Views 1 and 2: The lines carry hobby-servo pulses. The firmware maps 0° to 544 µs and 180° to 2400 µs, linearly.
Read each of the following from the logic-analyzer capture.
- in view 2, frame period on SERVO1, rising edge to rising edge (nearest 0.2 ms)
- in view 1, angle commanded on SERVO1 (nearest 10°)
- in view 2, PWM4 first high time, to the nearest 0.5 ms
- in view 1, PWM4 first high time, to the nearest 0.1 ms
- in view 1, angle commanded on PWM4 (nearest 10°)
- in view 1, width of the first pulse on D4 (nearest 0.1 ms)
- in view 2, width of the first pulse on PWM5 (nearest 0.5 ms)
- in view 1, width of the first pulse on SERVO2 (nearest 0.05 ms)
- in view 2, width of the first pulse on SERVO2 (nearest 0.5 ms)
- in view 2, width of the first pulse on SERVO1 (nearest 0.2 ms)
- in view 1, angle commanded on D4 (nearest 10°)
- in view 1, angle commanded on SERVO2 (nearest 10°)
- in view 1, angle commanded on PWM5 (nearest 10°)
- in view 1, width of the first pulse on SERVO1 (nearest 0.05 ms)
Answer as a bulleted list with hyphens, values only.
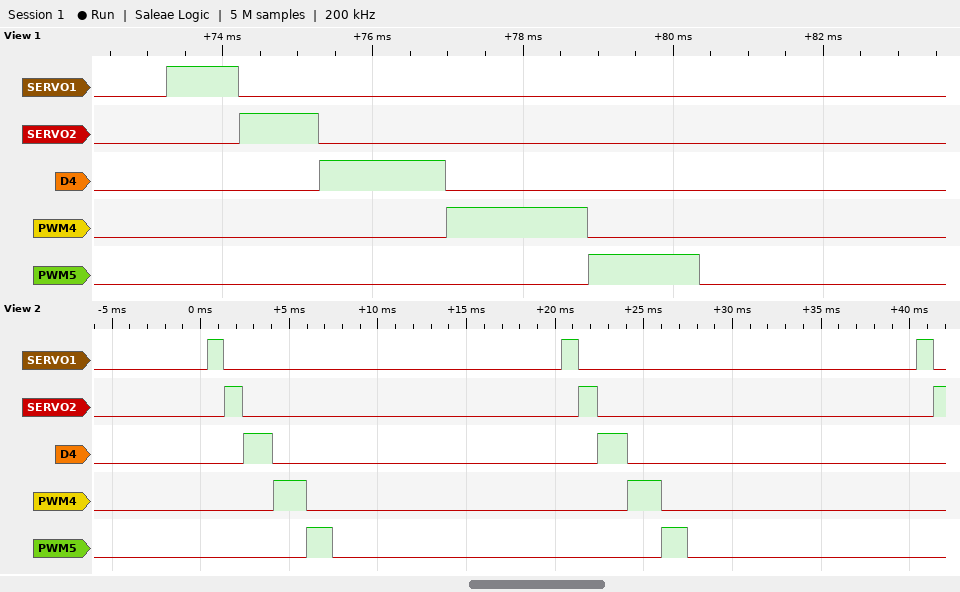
- 20.0 ms
- 40°
- 2.0 ms
- 1.9 ms
- 130°
- 1.7 ms
- 1.5 ms
- 1.05 ms
- 1.0 ms
- 1.0 ms
- 110°
- 50°
- 90°
- 0.95 ms
